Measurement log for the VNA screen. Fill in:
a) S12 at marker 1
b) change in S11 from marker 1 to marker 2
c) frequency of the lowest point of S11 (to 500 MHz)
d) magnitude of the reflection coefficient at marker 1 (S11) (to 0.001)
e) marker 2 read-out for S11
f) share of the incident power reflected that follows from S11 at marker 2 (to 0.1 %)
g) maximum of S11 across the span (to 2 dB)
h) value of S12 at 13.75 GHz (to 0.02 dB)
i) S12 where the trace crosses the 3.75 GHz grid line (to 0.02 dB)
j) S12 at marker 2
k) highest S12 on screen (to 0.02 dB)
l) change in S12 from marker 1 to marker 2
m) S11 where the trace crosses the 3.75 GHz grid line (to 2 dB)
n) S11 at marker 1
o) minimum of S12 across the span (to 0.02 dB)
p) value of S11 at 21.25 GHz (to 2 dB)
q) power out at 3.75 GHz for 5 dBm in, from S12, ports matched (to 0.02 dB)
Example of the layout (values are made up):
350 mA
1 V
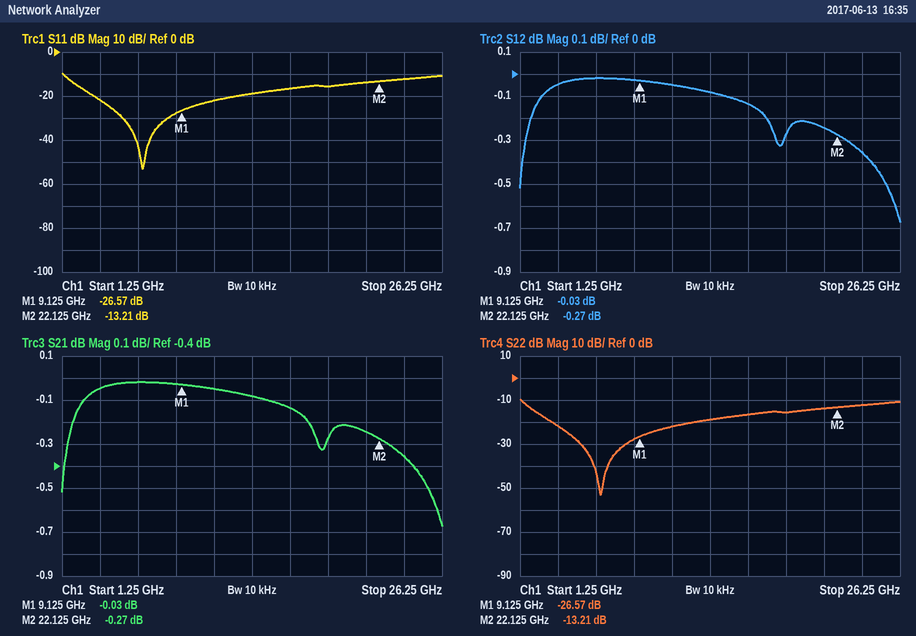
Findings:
-0.03 dB
13.36 dB
6.5 GHz
0.047
-13.21 dB
4.8 %
-10 dB
-0.08 dB
-0.04 dB
-0.27 dB
-0.02 dB
-0.24 dB
-22 dB
-26.57 dB
-0.68 dB
-14 dB
4.96 dBm
